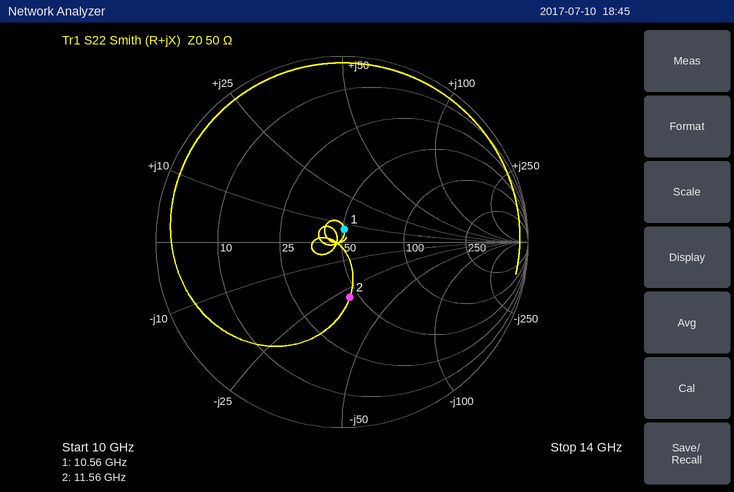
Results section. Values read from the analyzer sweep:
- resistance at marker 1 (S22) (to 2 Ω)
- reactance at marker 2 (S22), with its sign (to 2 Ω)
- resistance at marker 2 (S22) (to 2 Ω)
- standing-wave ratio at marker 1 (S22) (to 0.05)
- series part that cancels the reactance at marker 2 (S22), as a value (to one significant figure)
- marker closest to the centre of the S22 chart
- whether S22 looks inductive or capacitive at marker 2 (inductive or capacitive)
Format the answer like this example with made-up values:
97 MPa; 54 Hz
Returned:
50 Ω; -30 Ω; 46 Ω; 1.15; 400 pH; marker 1; capacitive
